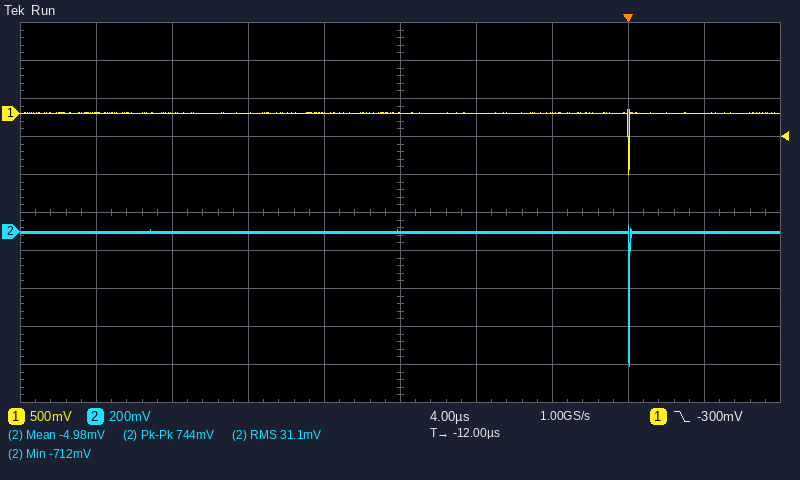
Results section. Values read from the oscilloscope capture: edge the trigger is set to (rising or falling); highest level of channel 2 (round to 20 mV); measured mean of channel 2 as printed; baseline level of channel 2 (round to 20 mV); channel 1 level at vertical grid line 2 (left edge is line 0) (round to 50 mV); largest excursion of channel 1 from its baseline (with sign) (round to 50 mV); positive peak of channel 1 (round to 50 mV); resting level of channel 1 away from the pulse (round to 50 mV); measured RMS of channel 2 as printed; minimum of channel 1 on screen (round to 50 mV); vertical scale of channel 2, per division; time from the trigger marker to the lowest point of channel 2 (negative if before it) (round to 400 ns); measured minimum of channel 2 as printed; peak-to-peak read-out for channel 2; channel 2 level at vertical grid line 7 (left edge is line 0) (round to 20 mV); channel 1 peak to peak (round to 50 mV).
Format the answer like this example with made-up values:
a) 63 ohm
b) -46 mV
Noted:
a) falling
b) 40 mV
c) -4.98 mV
d) 0 mV
e) 0 mV
f) -800 mV
g) 50 mV
h) 0 mV
i) 31.1 mV
j) -800 mV
k) 200 mV
l) 0.0 µs
m) -712 mV
n) 744 mV
o) 0 mV
p) 850 mV
